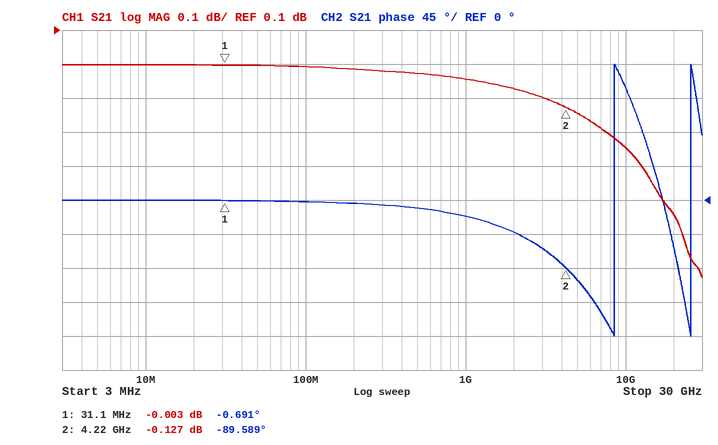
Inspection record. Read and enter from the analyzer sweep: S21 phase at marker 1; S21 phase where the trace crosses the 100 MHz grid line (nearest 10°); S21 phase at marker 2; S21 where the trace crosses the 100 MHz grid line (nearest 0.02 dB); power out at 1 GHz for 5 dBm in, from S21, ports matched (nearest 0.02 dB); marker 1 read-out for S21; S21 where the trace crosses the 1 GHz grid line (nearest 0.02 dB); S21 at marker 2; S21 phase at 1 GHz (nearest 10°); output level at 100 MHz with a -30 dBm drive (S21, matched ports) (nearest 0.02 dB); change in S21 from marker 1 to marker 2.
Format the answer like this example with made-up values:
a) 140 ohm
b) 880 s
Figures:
a) -0.691°
b) 0°
c) -89.589°
d) 0.00 dB
e) 4.96 dBm
f) -0.003 dB
g) -0.04 dB
h) -0.127 dB
i) -20°
j) -30.00 dBm
k) -0.124 dB
